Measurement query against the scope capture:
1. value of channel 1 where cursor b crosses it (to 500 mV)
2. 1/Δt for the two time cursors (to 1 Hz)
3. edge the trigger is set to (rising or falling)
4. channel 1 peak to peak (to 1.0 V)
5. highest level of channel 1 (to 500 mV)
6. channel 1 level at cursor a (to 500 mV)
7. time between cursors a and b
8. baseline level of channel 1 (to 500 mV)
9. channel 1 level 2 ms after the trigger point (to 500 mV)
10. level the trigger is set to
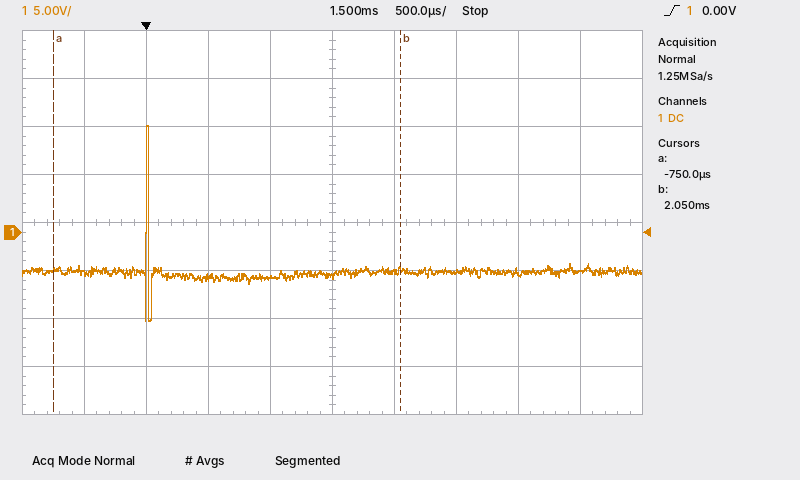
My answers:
-4.0 V
357 Hz
rising
20.0 V
11.0 V
-4.0 V
2.80 ms
-4.0 V
-4.0 V
0.00 V
